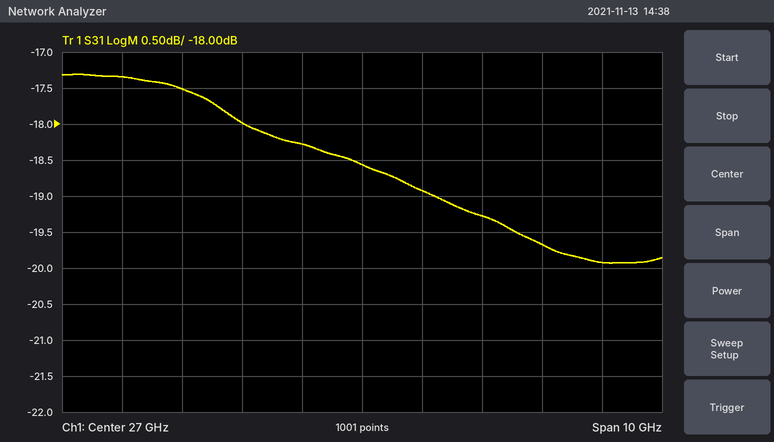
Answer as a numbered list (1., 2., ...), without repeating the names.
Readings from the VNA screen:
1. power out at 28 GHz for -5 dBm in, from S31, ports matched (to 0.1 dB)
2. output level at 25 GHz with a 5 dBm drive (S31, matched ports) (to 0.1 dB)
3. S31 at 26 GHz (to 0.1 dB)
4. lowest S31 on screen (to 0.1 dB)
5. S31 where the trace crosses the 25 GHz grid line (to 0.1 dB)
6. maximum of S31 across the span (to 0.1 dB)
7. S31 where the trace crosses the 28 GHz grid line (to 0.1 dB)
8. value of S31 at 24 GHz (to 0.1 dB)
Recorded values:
1. -23.9 dBm
2. -13.0 dBm
3. -18.3 dB
4. -19.9 dB
5. -18.0 dB
6. -17.3 dB
7. -18.9 dB
8. -17.5 dB
